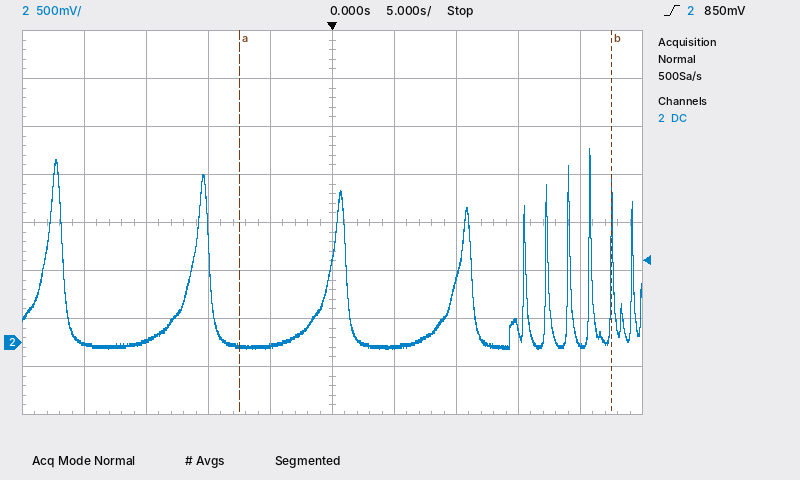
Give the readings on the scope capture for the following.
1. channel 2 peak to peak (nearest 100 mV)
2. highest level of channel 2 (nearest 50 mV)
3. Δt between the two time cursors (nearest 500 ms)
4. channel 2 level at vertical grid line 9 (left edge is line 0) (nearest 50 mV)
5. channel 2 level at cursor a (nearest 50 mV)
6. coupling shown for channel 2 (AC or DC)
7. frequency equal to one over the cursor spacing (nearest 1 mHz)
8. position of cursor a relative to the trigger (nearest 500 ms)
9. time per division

2.10 V
2.00 V
30.0 s
0 mV
-50 mV
DC
33 mHz
-7.5 s
5 s
